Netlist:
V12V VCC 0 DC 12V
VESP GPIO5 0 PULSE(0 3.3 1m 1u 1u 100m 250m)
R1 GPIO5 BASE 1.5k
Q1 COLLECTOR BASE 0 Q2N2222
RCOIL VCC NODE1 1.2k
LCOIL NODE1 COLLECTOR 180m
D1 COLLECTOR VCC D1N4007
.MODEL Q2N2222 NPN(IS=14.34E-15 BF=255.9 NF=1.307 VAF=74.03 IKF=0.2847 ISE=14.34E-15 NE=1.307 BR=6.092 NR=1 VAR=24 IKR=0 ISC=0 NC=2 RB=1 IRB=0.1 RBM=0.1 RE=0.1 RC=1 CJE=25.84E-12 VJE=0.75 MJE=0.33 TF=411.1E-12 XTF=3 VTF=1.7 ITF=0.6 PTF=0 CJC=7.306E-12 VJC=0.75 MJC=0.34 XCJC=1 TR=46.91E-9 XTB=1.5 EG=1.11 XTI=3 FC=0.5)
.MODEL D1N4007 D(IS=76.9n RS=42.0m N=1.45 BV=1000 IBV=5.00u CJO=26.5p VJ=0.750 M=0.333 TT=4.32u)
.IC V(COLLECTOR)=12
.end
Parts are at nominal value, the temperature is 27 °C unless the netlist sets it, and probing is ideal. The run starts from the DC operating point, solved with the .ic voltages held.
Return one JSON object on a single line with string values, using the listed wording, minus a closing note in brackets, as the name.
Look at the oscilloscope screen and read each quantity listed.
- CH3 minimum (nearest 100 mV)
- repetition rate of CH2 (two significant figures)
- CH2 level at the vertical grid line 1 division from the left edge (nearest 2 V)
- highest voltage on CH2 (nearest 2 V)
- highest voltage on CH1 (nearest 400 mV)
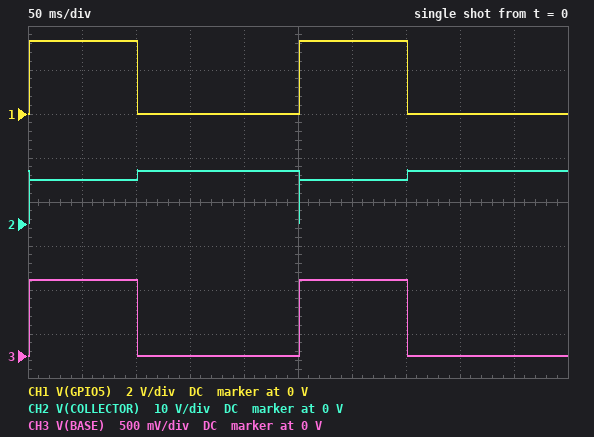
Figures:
{"CH3 minimum": "0 V", "repetition rate of CH2": "4.0 Hz", "CH2 level at the vertical grid line 1 division from the left edge": "10 V", "highest voltage on CH2": "12 V", "highest voltage on CH1": "3.2 V"}
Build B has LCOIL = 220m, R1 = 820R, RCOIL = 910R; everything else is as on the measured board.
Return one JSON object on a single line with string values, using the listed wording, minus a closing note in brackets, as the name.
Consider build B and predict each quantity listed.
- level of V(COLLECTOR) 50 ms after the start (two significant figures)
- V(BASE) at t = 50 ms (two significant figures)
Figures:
{"level of V(COLLECTOR) 50 ms after the start": "9.2 V", "V(BASE) at t = 50 ms": "880 mV"}
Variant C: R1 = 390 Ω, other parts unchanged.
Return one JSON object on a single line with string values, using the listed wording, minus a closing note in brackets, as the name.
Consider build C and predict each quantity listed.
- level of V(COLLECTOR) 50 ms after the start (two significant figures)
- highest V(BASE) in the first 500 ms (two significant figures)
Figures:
{"level of V(COLLECTOR) 50 ms after the start": "4.7 V", "highest V(BASE) in the first 500 ms": "910 mV"}
